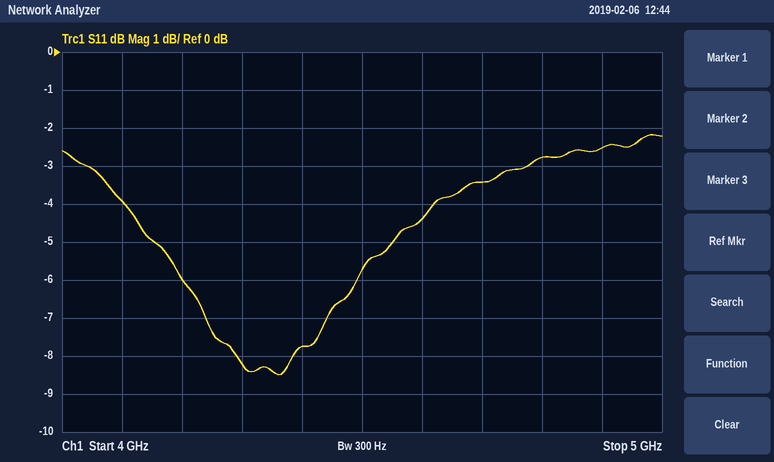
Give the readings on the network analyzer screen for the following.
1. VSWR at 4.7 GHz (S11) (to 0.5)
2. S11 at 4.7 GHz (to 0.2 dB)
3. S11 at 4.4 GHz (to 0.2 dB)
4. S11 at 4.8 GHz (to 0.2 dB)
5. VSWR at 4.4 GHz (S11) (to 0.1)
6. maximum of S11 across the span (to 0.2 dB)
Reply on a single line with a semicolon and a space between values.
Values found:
5.0; -3.4 dB; -7.8 dB; -2.8 dB; 2.4; -2.2 dB
